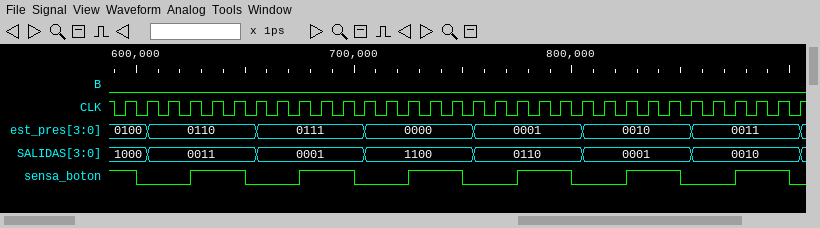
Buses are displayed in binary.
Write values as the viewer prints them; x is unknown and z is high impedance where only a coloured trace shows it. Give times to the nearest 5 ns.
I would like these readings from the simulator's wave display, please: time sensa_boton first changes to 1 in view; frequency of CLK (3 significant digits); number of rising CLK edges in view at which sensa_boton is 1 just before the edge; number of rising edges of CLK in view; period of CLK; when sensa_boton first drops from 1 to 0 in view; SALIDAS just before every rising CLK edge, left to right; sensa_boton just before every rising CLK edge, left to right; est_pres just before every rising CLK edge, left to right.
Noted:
625 ns
100 MHz
13
32
10 ns
600 ns
1000, 1000, 0011, 0011, 0011, 0011, 0011, 0001, 0001, 0001, 0001, 0001, 1100, 1100, 1100, 1100, 1100, 0110, 0110, 0110, 0110, 0110, 0001, 0001, 0001, 0001, 0001, 0010, 0010, 0010, 0010, 0010
1 0 0 0 1 1 0 0 0 1 1 0 0 0 1 1 0 0 0 1 1 0 0 0 1 1 0 0 0 1 1 0
0100, 0100, 0110, 0110, 0110, 0110, 0110, 0111, 0111, 0111, 0111, 0111, 0000, 0000, 0000, 0000, 0000, 0001, 0001, 0001, 0001, 0001, 0010, 0010, 0010, 0010, 0010, 0011, 0011, 0011, 0011, 0011
